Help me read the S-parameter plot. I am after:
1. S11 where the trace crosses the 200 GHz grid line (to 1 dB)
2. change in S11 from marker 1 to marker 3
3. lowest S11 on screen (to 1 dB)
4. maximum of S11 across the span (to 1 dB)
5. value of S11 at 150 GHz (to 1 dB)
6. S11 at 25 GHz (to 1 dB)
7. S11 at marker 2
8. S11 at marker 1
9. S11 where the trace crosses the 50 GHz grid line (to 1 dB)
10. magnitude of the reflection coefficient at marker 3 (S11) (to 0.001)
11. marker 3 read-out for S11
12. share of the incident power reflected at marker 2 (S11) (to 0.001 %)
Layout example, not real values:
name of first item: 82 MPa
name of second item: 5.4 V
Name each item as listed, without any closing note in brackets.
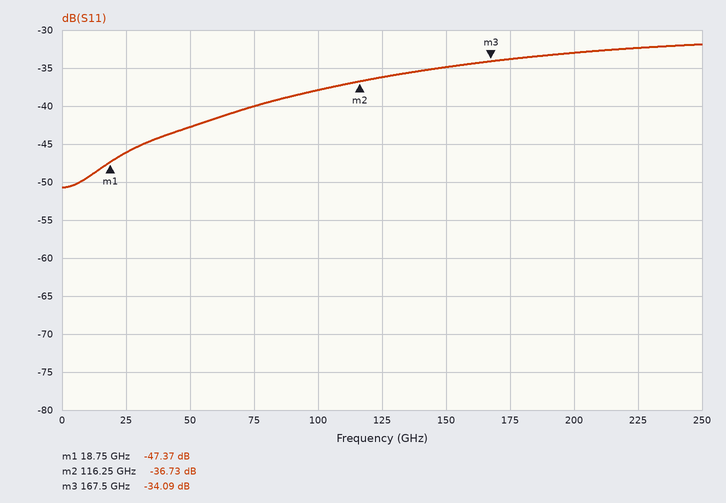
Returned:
S11 where the trace crosses the 200 GHz grid line: -33 dB
change in S11 from marker 1 to marker 3: 13.28 dB
lowest S11 on screen: -51 dB
maximum of S11 across the span: -32 dB
value of S11 at 150 GHz: -35 dB
S11 at 25 GHz: -46 dB
S11 at marker 2: -36.73 dB
S11 at marker 1: -47.37 dB
S11 where the trace crosses the 50 GHz grid line: -43 dB
magnitude of the reflection coefficient at marker 3 (S11): 0.020
marker 3 read-out for S11: -34.09 dB
share of the incident power reflected at marker 2 (S11): 0.021 %
